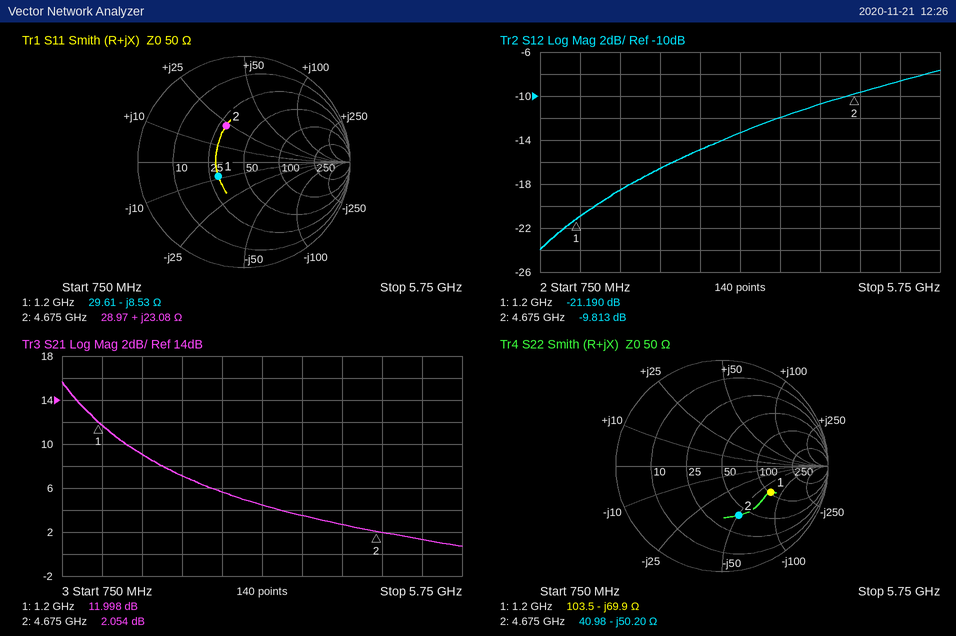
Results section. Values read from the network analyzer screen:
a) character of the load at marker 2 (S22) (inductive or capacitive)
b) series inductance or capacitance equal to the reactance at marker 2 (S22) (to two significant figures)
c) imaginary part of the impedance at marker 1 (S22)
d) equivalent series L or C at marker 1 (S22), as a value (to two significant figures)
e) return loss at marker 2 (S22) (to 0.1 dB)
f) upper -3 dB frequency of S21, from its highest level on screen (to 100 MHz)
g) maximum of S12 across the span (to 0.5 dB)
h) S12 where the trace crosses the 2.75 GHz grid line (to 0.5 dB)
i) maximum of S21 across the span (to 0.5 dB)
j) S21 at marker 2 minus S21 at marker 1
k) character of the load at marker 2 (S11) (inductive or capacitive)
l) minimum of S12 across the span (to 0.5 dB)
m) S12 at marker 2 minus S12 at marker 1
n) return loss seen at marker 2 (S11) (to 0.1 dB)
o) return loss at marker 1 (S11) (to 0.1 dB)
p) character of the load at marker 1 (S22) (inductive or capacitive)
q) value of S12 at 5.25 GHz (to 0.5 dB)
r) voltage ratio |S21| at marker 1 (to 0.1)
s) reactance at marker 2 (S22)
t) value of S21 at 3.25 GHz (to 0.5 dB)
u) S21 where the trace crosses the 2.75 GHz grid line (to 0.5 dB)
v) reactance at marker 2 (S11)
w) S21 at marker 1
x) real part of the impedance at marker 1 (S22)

capacitive
680 fF
-69.9 Ω
1.9 pF
6.2 dB
1.1 GHz
-7.5 dB
-15.0 dB
15.5 dB
-9.944 dB
inductive
-24.0 dB
11.377 dB
8.4 dB
11.2 dB
capacitive
-8.5 dB
4.0
-50.20 Ω
4.5 dB
5.5 dB
+23.08 Ω
11.998 dB
103.5 Ω
